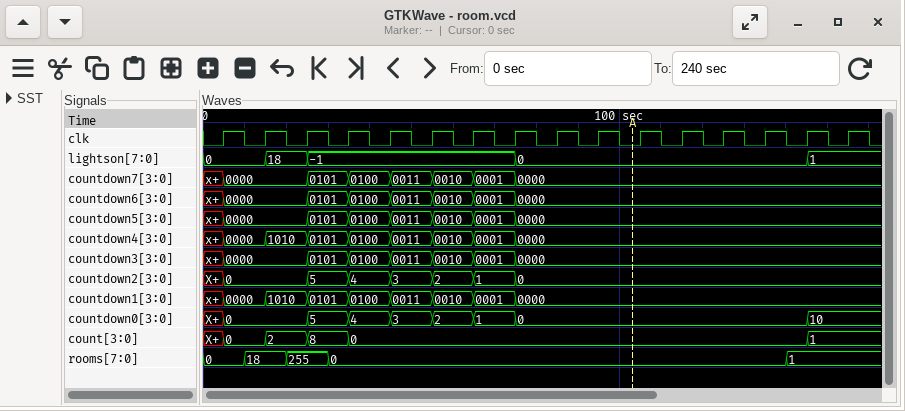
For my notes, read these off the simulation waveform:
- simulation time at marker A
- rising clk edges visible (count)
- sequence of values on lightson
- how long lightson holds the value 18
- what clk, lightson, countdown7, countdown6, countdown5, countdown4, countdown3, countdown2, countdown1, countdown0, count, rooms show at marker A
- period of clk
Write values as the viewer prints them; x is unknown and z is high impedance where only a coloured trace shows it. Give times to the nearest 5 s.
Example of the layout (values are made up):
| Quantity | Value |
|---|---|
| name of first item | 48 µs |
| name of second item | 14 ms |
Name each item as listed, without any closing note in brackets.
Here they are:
| Quantity | Value |
|---|---|
| simulation time at marker A | 105 s |
| rising clk edges visible | 16 |
| sequence of values on lightson | 0, 18, -1, 0, 1 |
| how long lightson holds the value 18 | 10 s |
| what clk, lightson, countdown7, countdown6, countdown5, countdown4, countdown3, countdown2, countdown1, countdown0, count, rooms show at marker A | clk=0, lightson=0, countdown7=0000, countdown6=0000, countdown5=0000, countdown4=0000, countdown3=0000, countdown2=0, countdown1=0000, countdown0=0, count=0, rooms=0 |
| period of clk | 10 s |
